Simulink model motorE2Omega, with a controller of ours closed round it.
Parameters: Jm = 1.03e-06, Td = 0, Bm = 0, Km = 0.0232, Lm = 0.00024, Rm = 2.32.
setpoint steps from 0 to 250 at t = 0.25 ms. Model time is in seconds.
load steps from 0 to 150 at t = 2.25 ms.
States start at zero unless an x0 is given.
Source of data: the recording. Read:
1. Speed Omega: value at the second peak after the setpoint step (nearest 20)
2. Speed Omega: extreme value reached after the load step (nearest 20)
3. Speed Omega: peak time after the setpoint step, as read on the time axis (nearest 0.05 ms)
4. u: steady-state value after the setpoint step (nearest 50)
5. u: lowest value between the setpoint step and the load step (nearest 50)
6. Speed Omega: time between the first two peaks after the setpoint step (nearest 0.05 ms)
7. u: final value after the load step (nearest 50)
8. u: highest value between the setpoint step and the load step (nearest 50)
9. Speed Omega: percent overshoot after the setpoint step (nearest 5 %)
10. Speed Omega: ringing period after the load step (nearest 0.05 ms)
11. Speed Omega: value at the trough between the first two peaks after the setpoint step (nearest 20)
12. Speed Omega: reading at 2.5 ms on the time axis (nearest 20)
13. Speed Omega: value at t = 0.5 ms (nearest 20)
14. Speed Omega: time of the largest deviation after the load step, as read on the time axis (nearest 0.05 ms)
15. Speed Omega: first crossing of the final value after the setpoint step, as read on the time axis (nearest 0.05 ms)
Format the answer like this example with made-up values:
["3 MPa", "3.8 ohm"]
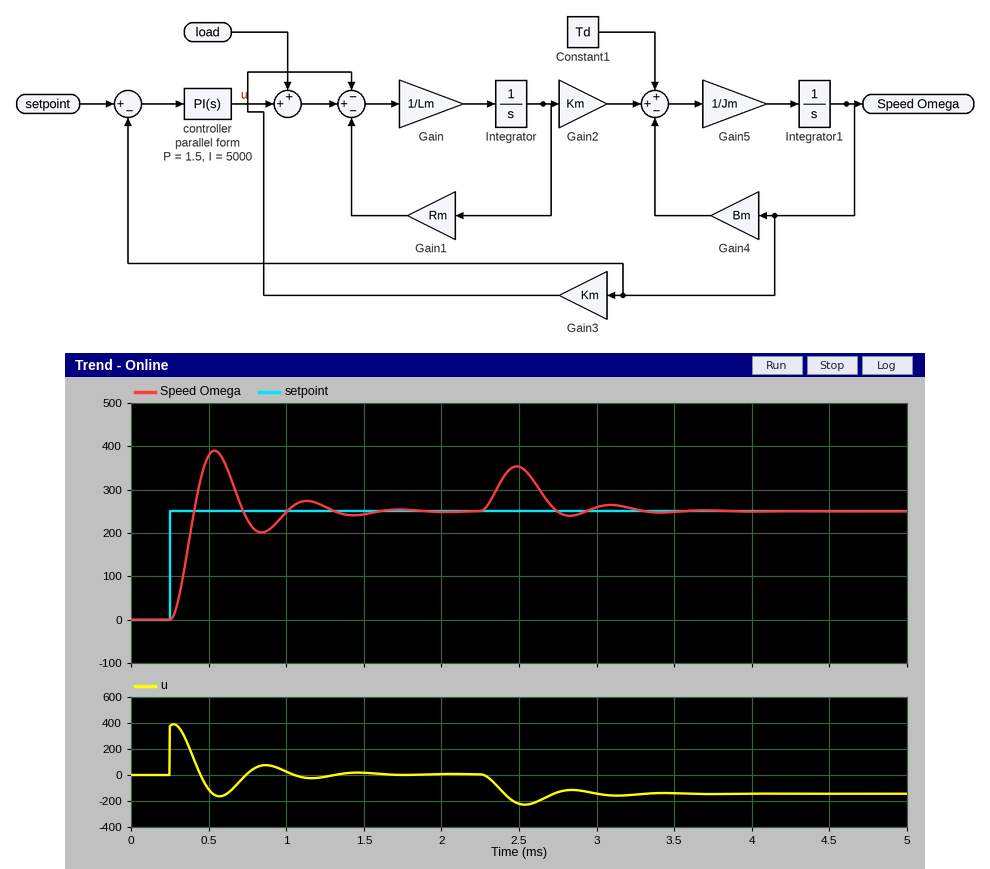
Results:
["280", "360", "0.55 ms", "0", "-150", "0.60 ms", "-150", "400", "55 %", "0.60 ms", "200", "360", "380", "2.50 ms", "0.40 ms"]
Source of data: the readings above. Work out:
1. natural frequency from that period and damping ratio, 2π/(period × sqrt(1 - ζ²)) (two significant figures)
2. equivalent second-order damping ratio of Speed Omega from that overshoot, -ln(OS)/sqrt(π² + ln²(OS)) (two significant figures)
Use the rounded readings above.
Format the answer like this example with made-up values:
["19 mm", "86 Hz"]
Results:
["11 rad/ms", "0.19"]
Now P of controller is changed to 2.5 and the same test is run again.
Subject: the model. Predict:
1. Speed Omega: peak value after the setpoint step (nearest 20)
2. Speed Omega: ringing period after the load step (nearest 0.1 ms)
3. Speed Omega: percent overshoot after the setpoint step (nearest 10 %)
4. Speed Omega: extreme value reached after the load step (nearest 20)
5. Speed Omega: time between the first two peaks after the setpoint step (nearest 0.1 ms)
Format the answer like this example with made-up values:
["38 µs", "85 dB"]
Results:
["380", "0.4 ms", "50 %", "320", "0.4 ms"]
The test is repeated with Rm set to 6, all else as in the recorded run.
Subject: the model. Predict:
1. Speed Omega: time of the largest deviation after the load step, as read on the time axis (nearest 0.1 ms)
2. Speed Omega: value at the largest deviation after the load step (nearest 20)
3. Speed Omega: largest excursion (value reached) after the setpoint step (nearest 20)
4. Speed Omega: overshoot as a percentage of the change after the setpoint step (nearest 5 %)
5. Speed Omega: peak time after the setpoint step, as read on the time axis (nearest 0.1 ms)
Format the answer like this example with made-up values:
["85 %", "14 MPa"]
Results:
["2.5 ms", "320", "320", "30 %", "0.7 ms"]
